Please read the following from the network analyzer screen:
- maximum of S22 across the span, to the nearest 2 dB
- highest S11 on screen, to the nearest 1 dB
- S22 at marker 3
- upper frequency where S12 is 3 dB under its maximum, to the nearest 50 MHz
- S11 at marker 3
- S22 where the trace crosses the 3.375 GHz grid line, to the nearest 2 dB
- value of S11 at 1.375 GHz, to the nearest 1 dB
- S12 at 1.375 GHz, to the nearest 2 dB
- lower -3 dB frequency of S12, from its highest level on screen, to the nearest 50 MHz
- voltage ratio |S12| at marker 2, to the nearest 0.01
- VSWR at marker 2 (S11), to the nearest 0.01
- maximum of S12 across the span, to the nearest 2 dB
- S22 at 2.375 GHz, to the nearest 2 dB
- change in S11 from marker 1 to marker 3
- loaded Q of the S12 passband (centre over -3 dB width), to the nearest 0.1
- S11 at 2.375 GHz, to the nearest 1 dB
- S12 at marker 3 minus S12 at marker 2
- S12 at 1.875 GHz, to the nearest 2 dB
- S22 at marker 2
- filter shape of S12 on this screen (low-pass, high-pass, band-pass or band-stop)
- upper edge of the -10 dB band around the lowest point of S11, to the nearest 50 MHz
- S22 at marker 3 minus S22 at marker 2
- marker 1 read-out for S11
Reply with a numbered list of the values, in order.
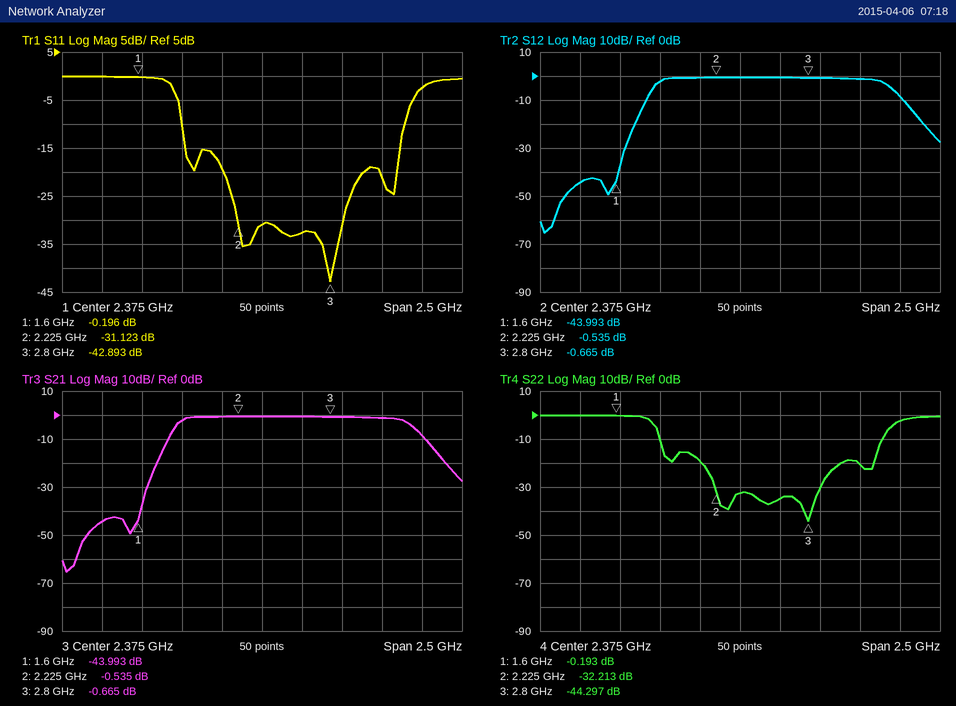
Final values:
1. 0 dB
2. 0 dB
3. -44.297 dB
4. 3.30 GHz
5. -42.893 dB
6. -2 dB
7. 0 dB
8. -44 dB
9. 1.85 GHz
10. 0.94
11. 1.06
12. 0 dB
13. -32 dB
14. -42.697 dB
15. 1.8
16. -31 dB
17. -0.130 dB
18. -2 dB
19. -32.213 dB
20. band-pass
21. 3.25 GHz
22. -12.084 dB
23. -0.196 dB
